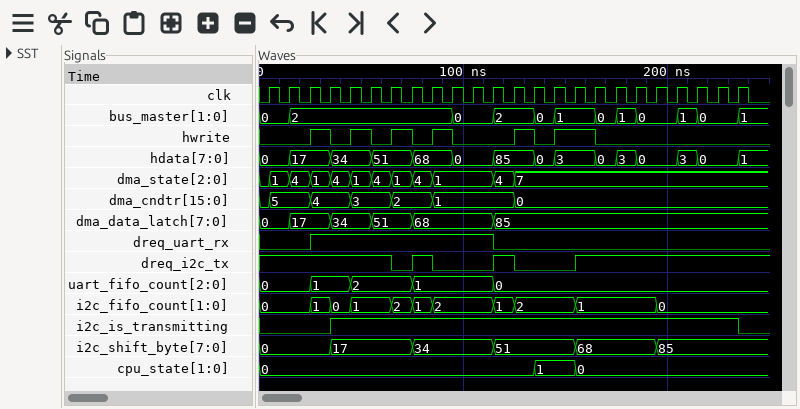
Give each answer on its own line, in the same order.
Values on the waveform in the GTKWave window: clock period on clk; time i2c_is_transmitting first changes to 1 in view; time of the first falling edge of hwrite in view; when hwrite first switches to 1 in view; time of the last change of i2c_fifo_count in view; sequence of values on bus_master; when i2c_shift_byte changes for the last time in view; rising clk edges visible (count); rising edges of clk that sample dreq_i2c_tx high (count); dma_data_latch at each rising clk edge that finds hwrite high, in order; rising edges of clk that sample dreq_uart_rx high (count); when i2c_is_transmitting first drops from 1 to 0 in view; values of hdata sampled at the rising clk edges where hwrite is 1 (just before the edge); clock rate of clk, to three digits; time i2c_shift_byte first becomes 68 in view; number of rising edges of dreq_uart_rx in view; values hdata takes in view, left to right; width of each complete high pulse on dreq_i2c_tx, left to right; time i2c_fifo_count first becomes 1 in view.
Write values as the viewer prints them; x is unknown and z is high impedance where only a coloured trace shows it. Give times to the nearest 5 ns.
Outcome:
10 ns
35 ns
35 ns
25 ns
195 ns
0, 2, 0, 2, 0, 1, 0, 1, 0, 1, 0, 1
195 ns
24
17
17, 34, 51, 68, 85, 85, 85
9
235 ns
17, 34, 51, 68, 85, 3, 3
100 MHz
155 ns
1
0, 17, 34, 51, 68, 0, 85, 0, 3, 0, 3, 0, 3, 0, 1
10 ns, 10 ns
25 ns
